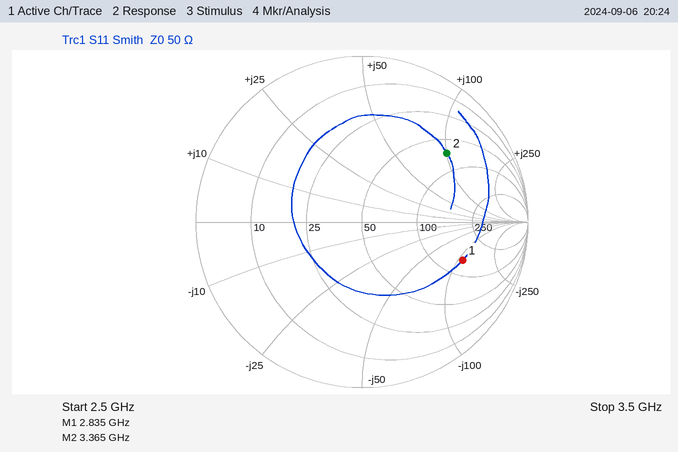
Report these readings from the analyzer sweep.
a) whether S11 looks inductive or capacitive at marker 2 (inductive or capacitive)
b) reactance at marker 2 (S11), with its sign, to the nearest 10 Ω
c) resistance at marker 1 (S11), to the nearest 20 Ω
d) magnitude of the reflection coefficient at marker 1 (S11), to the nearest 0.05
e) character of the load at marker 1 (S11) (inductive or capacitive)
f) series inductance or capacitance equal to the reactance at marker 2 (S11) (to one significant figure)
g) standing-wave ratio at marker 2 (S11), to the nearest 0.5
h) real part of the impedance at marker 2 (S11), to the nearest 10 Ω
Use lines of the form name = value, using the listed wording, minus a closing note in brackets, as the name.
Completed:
whether S11 looks inductive or capacitive at marker 2 = inductive
reactance at marker 2 (S11), with its sign, to the nearest 10 Ω = +100 Ω
resistance at marker 1 (S11), to the nearest 20 Ω = 140 Ω
magnitude of the reflection coefficient at marker 1 (S11), to the nearest 0.05 = 0.65
character of the load at marker 1 (S11) = capacitive
series inductance or capacitance equal to the reactance at marker 2 (S11) = 5 nH
standing-wave ratio at marker 2 (S11), to the nearest 0.5 = 5.0
real part of the impedance at marker 2 (S11), to the nearest 10 Ω = 70 Ω
